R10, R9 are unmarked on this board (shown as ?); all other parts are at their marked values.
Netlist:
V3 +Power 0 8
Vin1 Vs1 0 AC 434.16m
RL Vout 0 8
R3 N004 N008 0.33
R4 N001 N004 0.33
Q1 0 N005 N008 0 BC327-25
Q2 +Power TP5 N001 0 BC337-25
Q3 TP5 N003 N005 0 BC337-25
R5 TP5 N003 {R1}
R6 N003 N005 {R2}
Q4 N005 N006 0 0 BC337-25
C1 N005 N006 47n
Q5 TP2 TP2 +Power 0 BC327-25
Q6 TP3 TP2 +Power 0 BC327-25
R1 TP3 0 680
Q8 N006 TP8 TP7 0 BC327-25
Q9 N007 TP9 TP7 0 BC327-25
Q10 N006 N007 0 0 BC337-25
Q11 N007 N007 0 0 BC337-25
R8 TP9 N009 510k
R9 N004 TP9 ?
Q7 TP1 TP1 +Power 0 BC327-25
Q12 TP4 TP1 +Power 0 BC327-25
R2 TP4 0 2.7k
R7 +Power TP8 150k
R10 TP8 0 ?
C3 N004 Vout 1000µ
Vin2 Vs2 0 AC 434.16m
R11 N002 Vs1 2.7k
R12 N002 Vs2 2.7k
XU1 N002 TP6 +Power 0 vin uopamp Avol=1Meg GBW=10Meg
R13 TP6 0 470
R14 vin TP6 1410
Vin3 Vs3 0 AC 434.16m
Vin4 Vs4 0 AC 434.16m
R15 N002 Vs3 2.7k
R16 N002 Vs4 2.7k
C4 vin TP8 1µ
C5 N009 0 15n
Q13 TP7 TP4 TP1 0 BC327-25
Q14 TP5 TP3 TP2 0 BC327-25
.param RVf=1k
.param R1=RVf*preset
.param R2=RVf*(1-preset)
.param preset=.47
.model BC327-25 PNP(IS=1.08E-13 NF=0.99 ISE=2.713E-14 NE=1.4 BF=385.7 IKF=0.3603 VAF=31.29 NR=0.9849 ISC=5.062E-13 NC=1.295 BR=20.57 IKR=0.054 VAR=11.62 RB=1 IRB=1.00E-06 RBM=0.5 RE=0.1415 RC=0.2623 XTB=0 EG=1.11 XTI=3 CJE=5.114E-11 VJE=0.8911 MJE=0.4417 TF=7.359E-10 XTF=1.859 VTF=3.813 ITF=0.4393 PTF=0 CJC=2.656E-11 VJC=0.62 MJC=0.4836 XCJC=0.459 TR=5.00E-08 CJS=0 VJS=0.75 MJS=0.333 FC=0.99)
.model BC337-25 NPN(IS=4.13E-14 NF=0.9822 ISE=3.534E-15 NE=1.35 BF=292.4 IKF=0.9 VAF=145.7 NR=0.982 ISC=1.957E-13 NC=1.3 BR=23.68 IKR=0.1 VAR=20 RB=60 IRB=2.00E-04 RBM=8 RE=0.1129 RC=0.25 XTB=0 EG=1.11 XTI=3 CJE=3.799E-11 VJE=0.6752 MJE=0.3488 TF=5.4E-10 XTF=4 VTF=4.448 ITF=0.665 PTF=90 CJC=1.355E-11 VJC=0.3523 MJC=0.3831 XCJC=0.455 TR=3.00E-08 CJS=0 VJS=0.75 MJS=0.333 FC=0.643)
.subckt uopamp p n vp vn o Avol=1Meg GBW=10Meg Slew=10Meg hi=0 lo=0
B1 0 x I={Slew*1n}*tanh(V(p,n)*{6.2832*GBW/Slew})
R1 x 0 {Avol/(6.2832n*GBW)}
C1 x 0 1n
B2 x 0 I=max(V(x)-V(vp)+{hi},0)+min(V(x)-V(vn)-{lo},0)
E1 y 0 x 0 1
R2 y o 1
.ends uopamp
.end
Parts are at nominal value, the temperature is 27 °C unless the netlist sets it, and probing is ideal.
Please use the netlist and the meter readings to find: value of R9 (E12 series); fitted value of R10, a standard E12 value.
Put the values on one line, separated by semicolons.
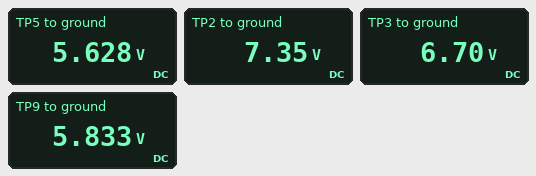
270 kΩ; 330 kΩ
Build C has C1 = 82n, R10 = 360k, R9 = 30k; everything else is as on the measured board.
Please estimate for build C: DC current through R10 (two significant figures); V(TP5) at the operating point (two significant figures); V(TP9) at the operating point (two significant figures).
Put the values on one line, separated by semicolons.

17 µA; 6.5 V; 6.0 V
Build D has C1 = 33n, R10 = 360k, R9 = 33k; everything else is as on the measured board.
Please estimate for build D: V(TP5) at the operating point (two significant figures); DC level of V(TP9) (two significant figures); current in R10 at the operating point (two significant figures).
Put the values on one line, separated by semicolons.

6.5 V; 6.0 V; 17 µA
